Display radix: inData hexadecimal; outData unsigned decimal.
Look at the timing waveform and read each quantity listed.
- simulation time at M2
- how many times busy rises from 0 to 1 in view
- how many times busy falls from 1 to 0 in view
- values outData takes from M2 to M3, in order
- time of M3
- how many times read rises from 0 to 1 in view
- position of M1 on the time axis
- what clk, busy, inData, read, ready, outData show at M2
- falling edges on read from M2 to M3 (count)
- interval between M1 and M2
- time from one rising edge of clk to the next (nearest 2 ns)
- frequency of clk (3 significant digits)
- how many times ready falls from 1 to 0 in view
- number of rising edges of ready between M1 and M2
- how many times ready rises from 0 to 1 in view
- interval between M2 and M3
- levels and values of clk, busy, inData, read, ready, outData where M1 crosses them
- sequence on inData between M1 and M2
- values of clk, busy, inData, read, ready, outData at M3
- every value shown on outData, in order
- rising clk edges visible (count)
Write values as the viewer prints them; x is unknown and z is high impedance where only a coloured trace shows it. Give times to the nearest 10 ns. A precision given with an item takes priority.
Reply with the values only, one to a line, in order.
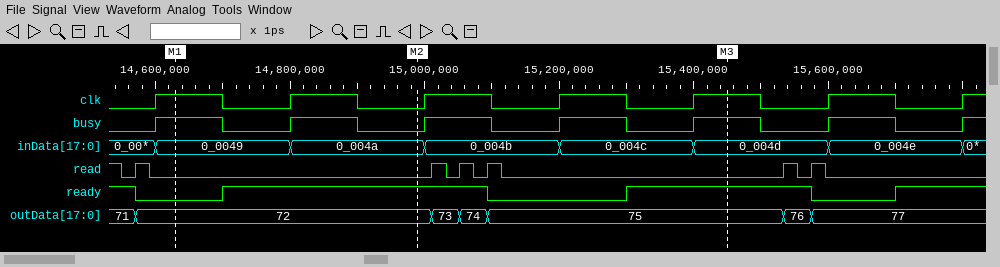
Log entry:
14990 ns
7
6
72, 73, 74, 75
15450 ns
6
14630 ns
clk=0, busy=0, inData=0_004a, read=0, ready=1, outData=72
3
360 ns
200 ns
5.00 MHz
3
1
3
460 ns
clk=1, busy=1, inData=0_0049, read=0, ready=0, outData=72
0_0049, 0_004a
clk=1, busy=1, inData=0_004d, read=0, ready=1, outData=75
71, 72, 73, 74, 75, 76, 77
7
